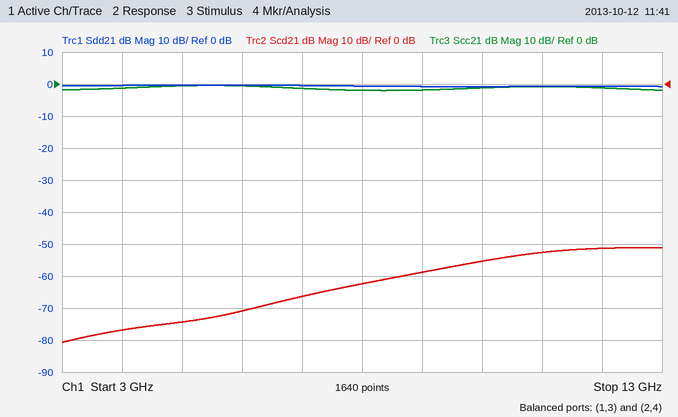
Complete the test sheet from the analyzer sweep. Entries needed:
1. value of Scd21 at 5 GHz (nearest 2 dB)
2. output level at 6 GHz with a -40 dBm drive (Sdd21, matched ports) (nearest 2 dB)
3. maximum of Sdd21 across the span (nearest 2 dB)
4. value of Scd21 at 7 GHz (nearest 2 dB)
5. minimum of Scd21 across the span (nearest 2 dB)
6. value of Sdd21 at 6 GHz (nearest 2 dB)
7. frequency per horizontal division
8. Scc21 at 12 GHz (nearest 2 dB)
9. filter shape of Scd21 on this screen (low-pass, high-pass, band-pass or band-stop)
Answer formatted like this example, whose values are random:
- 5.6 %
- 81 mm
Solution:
- -74 dB
- -40 dBm
- 0 dB
- -66 dB
- -80 dB
- 0 dB
- 1 GHz
- -2 dB
- high-pass
